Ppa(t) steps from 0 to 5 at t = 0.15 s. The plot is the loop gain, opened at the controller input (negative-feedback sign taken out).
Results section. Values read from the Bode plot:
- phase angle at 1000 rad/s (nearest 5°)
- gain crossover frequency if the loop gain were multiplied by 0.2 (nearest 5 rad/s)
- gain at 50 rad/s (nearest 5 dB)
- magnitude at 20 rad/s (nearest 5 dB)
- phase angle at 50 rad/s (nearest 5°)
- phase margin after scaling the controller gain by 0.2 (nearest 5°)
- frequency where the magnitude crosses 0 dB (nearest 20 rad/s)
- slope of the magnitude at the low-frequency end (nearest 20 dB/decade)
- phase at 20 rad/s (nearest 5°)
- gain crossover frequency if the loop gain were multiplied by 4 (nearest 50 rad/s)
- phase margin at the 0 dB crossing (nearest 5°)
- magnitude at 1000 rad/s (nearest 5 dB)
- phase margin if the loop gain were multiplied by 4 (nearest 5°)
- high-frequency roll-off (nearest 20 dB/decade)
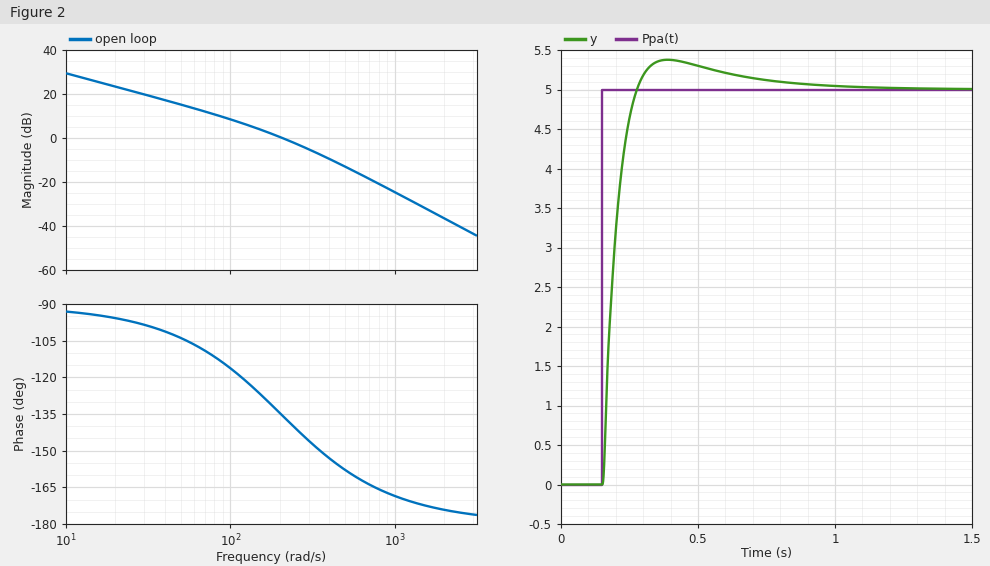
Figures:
-170°
55 rad/s
15 dB
25 dB
-105°
75°
200 rad/s
-20 dB/decade
-95°
450 rad/s
45°
-25 dB
25°
-40 dB/decade
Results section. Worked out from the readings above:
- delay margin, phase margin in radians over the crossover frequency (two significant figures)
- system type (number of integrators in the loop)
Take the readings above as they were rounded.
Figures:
0.0039 s
1
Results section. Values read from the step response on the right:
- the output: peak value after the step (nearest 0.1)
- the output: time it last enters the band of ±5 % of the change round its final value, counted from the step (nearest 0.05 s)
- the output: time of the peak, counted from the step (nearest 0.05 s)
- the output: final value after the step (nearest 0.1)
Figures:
5.4
0.40 s
0.25 s
5.0
